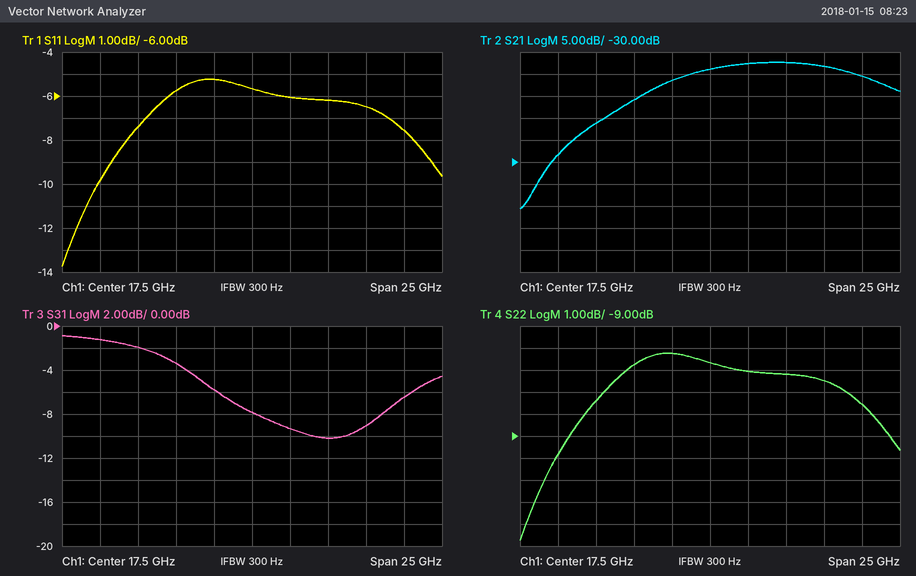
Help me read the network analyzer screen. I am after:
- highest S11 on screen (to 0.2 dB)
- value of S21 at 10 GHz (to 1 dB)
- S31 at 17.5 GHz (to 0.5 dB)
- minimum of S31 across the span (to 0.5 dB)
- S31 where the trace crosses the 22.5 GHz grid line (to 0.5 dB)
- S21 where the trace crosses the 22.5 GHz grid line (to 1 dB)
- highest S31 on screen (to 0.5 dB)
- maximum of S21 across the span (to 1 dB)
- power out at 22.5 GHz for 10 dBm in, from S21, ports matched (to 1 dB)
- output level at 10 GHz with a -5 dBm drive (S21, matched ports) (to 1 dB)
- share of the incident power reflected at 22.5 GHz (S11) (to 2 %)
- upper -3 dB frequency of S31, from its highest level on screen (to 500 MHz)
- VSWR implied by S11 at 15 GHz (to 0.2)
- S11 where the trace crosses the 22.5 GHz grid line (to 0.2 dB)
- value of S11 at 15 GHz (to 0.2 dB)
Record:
-5.2 dB
-21 dB
-8.0 dB
-10.0 dB
-10.0 dB
-7 dB
-1.0 dB
-7 dB
3 dBm
-26 dBm
24 %
13.0 GHz
3.4
-6.2 dB
-5.2 dB
